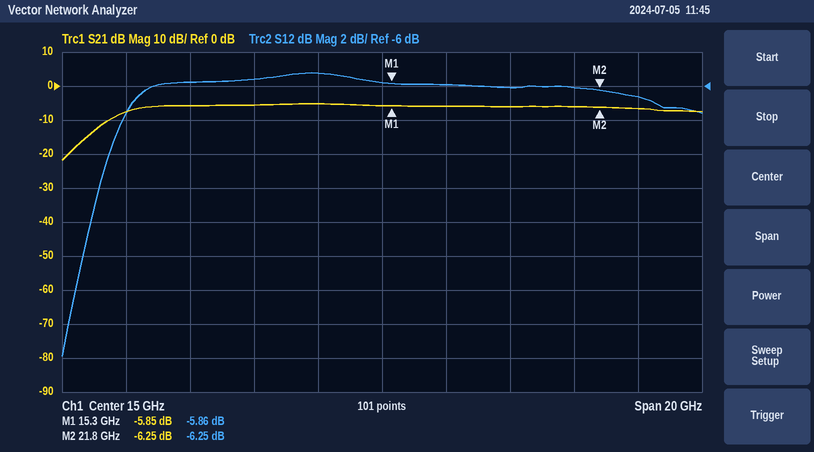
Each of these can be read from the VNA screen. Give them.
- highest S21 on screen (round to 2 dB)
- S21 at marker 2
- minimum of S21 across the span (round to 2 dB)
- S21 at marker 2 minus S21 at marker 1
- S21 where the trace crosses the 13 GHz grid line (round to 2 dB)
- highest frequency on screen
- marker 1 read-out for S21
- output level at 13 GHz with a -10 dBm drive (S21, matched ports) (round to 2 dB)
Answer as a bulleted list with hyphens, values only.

- -6 dB
- -6.25 dB
- -22 dB
- -0.40 dB
- -6 dB
- 25 GHz
- -5.85 dB
- -16 dBm
